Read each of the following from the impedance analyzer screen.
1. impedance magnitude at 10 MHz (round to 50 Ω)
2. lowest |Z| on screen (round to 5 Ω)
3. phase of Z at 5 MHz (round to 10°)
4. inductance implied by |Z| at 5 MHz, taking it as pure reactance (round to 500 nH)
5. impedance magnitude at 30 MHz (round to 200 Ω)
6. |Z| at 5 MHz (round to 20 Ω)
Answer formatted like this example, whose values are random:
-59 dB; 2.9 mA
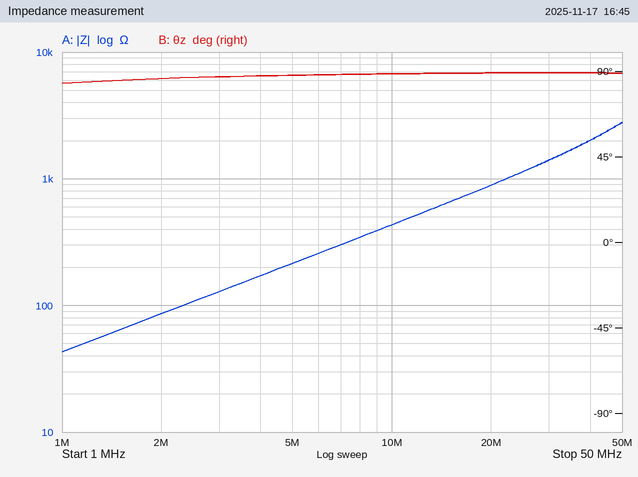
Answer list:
450 Ω; 45 Ω; 90°; 7.0 µH; 1.4 kΩ; 220 Ω
